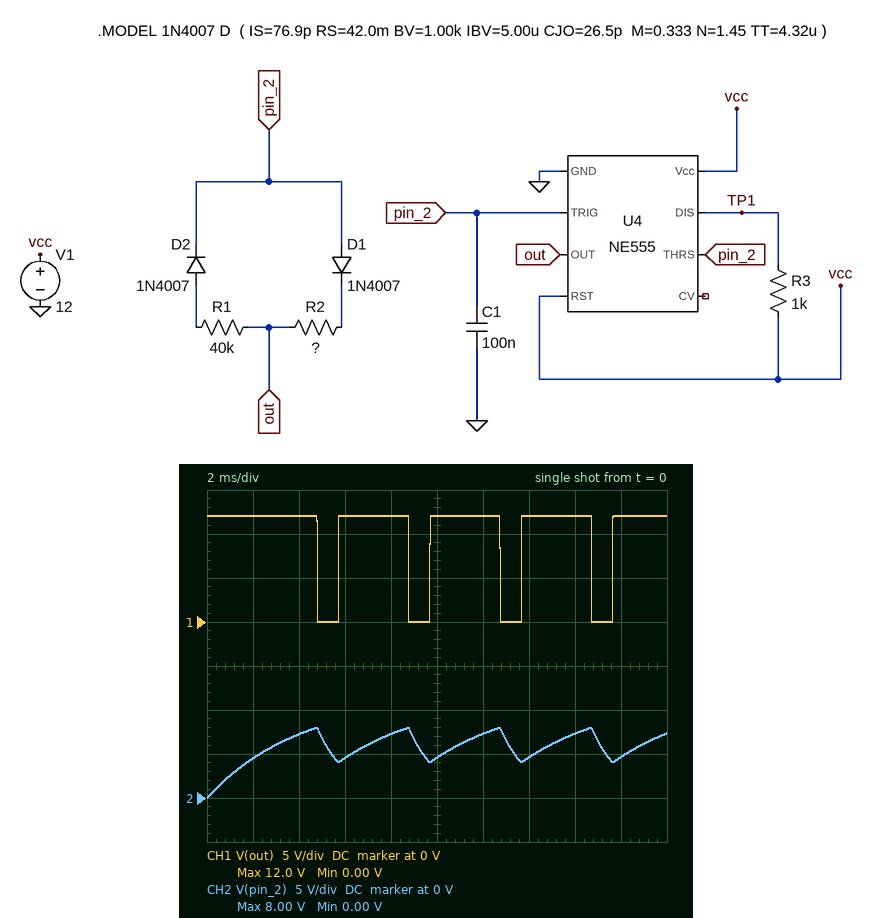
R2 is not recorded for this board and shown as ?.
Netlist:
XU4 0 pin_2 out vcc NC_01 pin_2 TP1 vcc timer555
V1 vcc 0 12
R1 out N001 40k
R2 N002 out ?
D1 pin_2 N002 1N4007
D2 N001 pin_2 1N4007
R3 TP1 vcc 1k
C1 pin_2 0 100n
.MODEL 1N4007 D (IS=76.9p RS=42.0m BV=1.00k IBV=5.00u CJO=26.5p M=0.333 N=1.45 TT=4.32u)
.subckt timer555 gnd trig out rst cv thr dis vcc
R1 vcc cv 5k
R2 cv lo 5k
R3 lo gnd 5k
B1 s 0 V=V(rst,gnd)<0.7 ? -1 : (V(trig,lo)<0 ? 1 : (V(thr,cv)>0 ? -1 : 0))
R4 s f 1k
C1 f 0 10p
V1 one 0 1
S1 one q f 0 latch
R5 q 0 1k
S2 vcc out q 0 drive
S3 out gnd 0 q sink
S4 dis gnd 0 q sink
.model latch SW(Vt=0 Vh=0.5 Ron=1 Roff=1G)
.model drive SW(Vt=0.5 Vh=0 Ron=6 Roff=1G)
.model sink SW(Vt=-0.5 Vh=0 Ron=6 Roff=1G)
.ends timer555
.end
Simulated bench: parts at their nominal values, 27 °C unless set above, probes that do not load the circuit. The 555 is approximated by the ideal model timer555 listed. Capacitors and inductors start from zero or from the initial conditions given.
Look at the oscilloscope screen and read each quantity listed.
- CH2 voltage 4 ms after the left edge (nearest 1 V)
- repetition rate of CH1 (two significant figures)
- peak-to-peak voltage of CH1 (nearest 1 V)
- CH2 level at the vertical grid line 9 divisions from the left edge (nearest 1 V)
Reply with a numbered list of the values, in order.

1. 7 V
2. 250 Hz
3. 12 V
4. 5 V
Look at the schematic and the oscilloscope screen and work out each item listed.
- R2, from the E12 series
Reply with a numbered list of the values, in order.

1. 12 kΩ
